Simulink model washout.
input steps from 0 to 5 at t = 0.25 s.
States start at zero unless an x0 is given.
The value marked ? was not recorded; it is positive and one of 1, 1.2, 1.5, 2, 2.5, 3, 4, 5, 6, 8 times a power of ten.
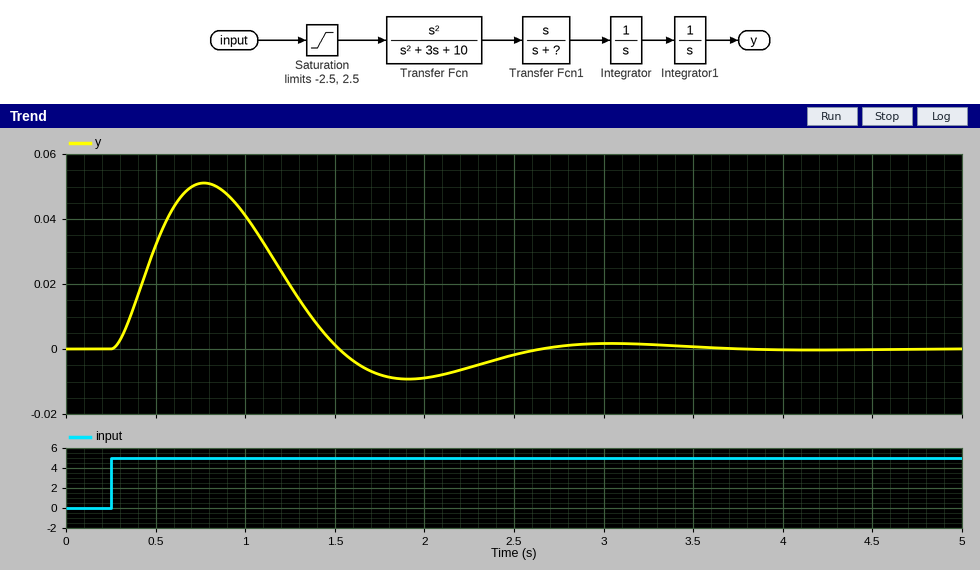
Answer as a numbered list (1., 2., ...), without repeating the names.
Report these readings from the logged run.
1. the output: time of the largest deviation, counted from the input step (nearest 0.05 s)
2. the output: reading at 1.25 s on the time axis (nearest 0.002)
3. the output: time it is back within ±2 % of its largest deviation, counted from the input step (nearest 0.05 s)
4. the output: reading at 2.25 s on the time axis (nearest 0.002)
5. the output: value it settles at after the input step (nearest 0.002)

1. 0.50 s
2. 0.020
3. 3.15 s
4. -0.006
5. 0.000
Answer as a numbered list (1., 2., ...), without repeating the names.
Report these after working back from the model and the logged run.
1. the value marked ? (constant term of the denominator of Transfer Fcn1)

1. 8
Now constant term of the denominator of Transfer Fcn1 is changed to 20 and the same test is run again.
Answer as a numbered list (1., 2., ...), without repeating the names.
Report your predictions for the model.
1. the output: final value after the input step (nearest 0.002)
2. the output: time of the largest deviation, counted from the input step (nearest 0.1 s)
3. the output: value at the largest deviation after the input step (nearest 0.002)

1. 0.000
2. 0.4 s
3. 0.022
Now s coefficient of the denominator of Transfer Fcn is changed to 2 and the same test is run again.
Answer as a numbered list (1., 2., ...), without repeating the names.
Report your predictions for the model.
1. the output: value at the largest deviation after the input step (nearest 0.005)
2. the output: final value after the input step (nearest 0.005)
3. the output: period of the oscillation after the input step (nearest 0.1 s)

1. 0.060
2. 0.000
3. 2.1 s
